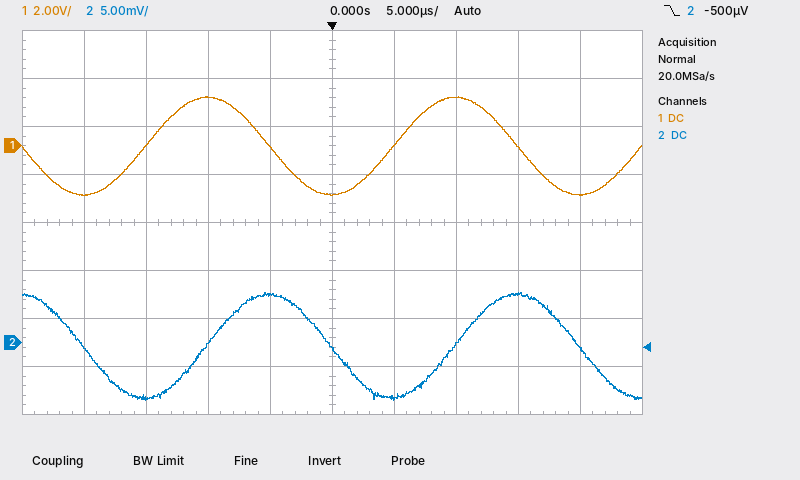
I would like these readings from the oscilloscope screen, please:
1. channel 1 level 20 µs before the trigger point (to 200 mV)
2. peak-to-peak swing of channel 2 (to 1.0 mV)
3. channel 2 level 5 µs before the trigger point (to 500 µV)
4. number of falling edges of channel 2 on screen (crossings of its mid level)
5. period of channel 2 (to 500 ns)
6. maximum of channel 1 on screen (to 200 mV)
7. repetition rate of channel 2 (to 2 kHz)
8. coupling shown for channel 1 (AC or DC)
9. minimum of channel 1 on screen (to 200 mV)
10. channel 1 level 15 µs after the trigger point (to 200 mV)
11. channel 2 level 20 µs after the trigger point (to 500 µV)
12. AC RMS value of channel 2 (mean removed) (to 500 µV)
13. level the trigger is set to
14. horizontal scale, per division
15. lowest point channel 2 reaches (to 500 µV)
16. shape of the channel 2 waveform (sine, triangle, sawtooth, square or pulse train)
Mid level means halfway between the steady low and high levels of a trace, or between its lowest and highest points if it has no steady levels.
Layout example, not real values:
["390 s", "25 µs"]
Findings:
["-2.0 V", "11.0 mV", "5.0 mV", "3", "20.0 µs", "2.0 V", "50 kHz", "DC", "-2.0 V", "0.0 V", "-500 µV", "4.0 mV", "-500 µV", "5 µs", "-6.0 mV", "sine"]
